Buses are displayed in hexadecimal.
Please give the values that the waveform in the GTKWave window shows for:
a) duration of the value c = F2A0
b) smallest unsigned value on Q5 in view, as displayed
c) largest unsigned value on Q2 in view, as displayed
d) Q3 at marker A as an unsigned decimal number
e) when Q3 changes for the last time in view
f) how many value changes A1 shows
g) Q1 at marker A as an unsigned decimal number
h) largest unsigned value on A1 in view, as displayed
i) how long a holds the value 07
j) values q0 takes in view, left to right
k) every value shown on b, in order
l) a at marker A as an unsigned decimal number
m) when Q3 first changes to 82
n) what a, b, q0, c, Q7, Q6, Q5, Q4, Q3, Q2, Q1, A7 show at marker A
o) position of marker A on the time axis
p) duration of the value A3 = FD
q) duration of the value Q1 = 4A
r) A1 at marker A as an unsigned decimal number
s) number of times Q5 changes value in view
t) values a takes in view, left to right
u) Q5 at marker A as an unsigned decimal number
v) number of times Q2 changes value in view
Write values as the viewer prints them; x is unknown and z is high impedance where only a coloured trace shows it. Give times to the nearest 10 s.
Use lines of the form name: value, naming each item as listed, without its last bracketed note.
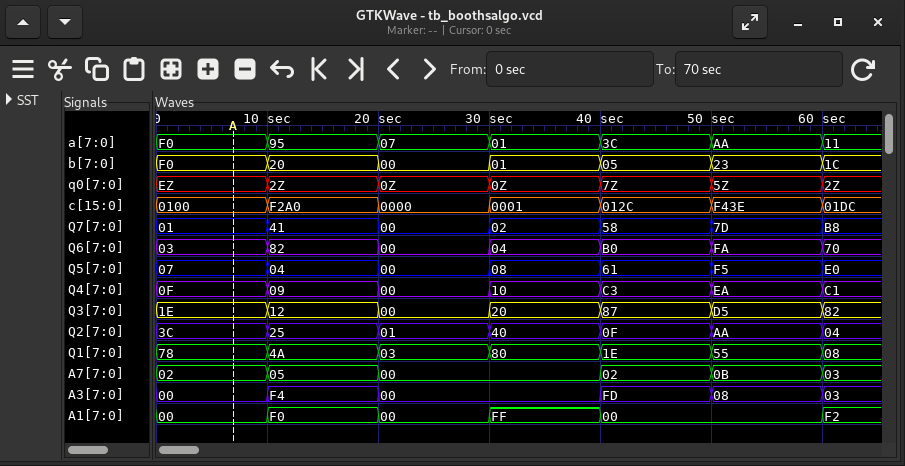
duration of the value c = F2A0: 10 s
smallest unsigned value on Q5 in view, as displayed: 00
largest unsigned value on Q2 in view, as displayed: AA
Q3 at marker A as an unsigned decimal number: 30
when Q3 changes for the last time in view: 60 s
how many value changes A1 shows: 5
Q1 at marker A as an unsigned decimal number: 120
largest unsigned value on A1 in view, as displayed: FF
how long a holds the value 07: 10 s
values q0 takes in view, left to right: EZ, 2Z, 0Z, 0Z, 7Z, 5Z, 2Z
every value shown on b, in order: F0, 20, 00, 01, 05, 23, 1C
a at marker A as an unsigned decimal number: 240
when Q3 first changes to 82: 60 s
what a, b, q0, c, Q7, Q6, Q5, Q4, Q3, Q2, Q1, A7 show at marker A: a=F0, b=F0, q0=EZ, c=0100, Q7=01, Q6=03, Q5=07, Q4=0F, Q3=1E, Q2=3C, Q1=78, A7=02
position of marker A on the time axis: 10 s
duration of the value A3 = FD: 10 s
duration of the value Q1 = 4A: 10 s
A1 at marker A as an unsigned decimal number: 0
number of times Q5 changes value in view: 6
values a takes in view, left to right: F0, 95, 07, 01, 3C, AA, 11
Q5 at marker A as an unsigned decimal number: 7
number of times Q2 changes value in view: 6
